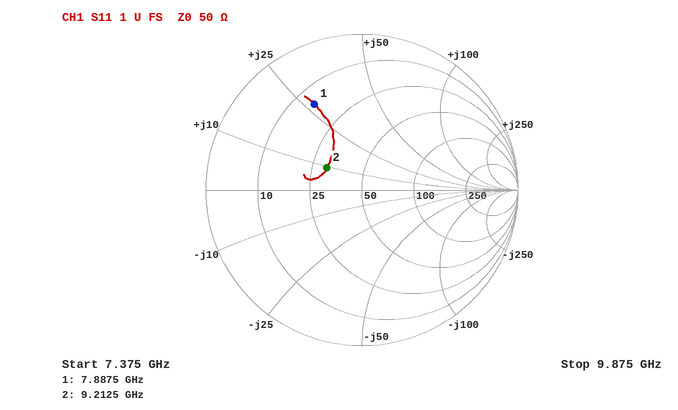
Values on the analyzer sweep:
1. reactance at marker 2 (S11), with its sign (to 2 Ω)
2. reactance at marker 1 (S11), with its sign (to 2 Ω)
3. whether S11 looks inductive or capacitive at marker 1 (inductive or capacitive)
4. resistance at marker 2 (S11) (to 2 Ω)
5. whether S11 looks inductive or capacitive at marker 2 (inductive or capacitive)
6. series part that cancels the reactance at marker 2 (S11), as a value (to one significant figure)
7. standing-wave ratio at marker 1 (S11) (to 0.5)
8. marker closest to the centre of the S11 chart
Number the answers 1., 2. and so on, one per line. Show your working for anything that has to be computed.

1. +10 Ω
2. +28 Ω
3. inductive
4. 30 Ω
5. inductive
6. C = 1/(2π × 9.2125 GHz × 10 Ω) ≈ 2 pF
7. 4.5
8. marker 2
